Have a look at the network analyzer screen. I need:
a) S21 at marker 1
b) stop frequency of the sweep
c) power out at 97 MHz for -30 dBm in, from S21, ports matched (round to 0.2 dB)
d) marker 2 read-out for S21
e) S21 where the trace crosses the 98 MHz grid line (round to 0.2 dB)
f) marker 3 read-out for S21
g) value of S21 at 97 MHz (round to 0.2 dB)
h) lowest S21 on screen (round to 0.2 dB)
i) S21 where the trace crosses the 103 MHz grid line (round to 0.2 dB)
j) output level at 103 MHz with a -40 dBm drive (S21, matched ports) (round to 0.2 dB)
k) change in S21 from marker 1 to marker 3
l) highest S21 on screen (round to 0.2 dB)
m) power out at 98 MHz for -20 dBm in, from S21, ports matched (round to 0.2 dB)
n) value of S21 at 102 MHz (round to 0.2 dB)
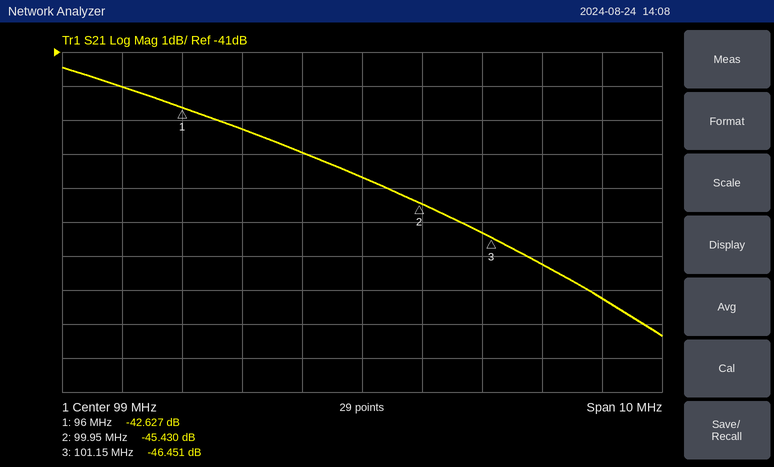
-42.627 dB
104 MHz
-73.2 dBm
-45.430 dB
-44.0 dB
-46.451 dB
-43.2 dB
-49.4 dB
-48.2 dB
-88.2 dBm
-3.824 dB
-41.4 dB
-64.0 dBm
-47.2 dB
